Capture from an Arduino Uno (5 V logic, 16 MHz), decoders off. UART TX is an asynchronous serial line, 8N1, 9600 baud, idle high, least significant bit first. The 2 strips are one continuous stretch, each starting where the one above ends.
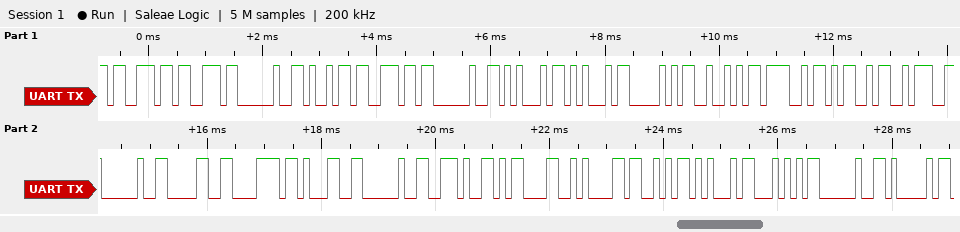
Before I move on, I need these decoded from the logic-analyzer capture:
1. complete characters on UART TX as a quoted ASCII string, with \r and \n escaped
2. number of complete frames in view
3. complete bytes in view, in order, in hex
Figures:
"ss in EEPROM: 0x1 .\r\nSET A"
26
73 73 20 69 6E 20 45 45 50 52 4F 4D 3A 20 30 78 31 20 2E 0D 0A 53 45 54 20 41
